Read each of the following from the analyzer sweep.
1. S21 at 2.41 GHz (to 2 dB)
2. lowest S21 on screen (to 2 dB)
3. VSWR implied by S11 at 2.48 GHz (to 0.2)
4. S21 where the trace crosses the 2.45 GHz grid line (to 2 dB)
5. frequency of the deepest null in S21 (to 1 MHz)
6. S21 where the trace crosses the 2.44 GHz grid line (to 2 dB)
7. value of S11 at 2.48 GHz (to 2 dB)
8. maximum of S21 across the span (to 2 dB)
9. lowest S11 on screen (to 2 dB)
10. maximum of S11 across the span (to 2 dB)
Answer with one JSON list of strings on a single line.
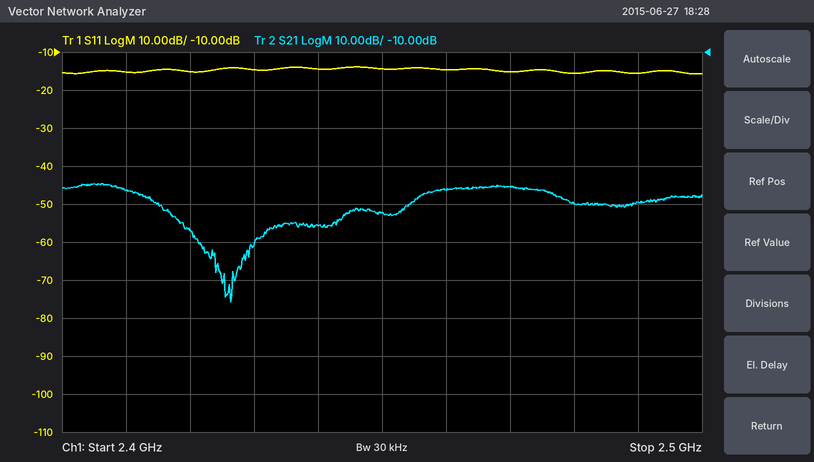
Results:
["-46 dB", "-76 dB", "1.4", "-52 dB", "2.426 GHz", "-56 dB", "-16 dB", "-44 dB", "-16 dB", "-14 dB"]
